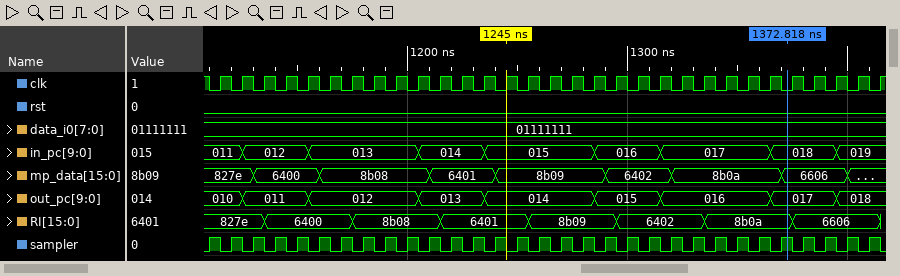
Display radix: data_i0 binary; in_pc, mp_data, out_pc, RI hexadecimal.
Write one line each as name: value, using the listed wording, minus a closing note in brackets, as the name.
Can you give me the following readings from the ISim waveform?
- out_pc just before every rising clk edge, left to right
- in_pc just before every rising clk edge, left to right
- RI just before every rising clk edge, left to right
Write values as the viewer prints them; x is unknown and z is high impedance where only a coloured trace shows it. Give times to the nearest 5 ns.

out_pc just before every rising clk edge, left to right: 010, 010, 011, 011, 011, 012, 012, 012, 012, 012, 013, 013, 013, 014, 014, 014, 014, 014, 015, 015, 015, 016, 016, 016, 016, 016, 017, 017, 017, 018, 018
in_pc just before every rising clk edge, left to right: 011, 011, 012, 012, 012, 013, 013, 013, 013, 013, 014, 014, 014, 015, 015, 015, 015, 015, 016, 016, 016, 017, 017, 017, 017, 017, 018, 018, 018, 019, 019
RI just before every rising clk edge, left to right: 827e, 827e, 827e, 6400, 6400, 6400, 6400, 8b08, 8b08, 8b08, 8b08, 6401, 6401, 6401, 6401, 8b09, 8b09, 8b09, 8b09, 6402, 6402, 6402, 6402, 8b0a, 8b0a, 8b0a, 8b0a, 6606, 6606, 6606, 6606
